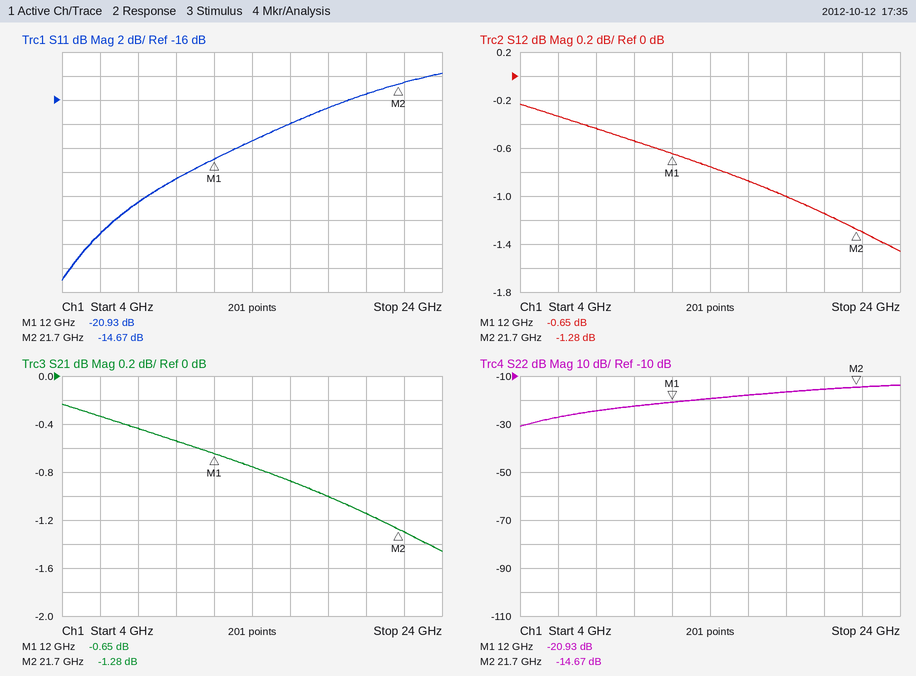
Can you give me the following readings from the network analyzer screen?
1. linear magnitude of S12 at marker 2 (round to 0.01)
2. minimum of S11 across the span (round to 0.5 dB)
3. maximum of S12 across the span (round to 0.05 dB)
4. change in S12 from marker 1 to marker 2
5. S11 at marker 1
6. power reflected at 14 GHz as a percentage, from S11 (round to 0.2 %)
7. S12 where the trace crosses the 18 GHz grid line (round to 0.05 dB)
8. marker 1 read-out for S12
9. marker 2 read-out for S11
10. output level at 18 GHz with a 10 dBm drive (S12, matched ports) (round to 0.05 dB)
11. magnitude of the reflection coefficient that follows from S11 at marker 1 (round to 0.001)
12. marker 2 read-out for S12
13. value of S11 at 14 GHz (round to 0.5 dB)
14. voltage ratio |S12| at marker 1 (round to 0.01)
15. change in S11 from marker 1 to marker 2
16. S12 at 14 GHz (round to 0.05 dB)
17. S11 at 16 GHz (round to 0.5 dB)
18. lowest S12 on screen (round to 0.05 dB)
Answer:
0.86
-31.0 dB
-0.25 dB
-0.63 dB
-20.93 dB
1.2 %
-1.00 dB
-0.65 dB
-14.67 dB
9.00 dBm
0.090
-1.28 dB
-19.5 dB
0.93
6.26 dB
-0.75 dB
-18.0 dB
-1.45 dB
